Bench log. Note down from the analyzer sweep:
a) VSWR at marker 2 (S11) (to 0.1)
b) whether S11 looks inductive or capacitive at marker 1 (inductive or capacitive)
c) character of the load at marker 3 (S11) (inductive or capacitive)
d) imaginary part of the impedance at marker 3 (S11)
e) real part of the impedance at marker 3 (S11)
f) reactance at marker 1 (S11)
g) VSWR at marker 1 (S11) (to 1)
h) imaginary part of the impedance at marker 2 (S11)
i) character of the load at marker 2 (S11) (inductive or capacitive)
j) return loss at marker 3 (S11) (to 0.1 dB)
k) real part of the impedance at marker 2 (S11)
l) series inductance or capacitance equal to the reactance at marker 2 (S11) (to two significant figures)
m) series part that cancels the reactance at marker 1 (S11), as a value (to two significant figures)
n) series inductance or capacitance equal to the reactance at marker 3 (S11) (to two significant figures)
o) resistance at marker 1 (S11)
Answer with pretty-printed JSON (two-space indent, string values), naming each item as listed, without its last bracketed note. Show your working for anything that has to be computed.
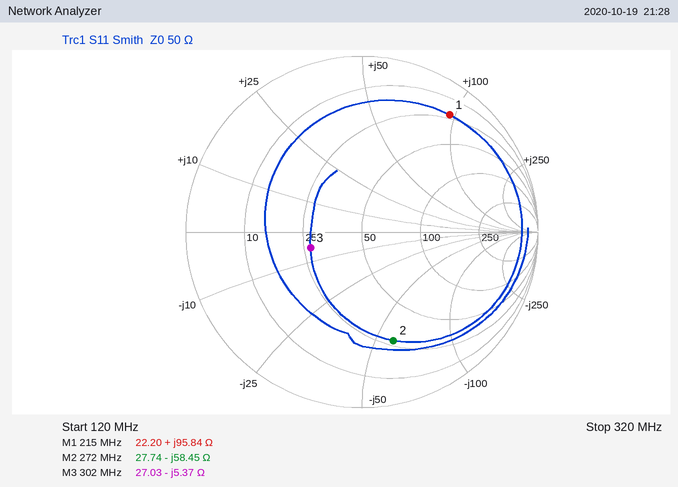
{
  "VSWR at marker 2 (S11)": "4.6",
  "whether S11 looks inductive or capacitive at marker 1": "inductive",
  "character of the load at marker 3 (S11)": "capacitive",
  "imaginary part of the impedance at marker 3": "-5.37 Ω",
  "real part of the impedance at marker 3": "27.03 Ω",
  "reactance at marker 1": "+95.84 Ω",
  "VSWR at marker 1 (S11)": "11",
  "imaginary part of the impedance at marker 2": "-58.45 Ω",
  "character of the load at marker 2 (S11)": "capacitive",
  "return loss at marker 3 (S11)": "10.3 dB",
  "real part of the impedance at marker 2": "27.74 Ω",
  "series inductance or capacitance equal to the reactance at marker 2 (S11)": "C = 1/(2π × 272 MHz × 58.45 Ω) ≈ 10 pF",
  "series part that cancels the reactance at marker 1 (S11), as a value": "C = 1/(2π × 215 MHz × 95.84 Ω) ≈ 7.7 pF",
  "series inductance or capacitance equal to the reactance at marker 3 (S11)": "C = 1/(2π × 302 MHz × 5.37 Ω) ≈ 98 pF",
  "resistance at marker 1": "22.20 Ω"
}
